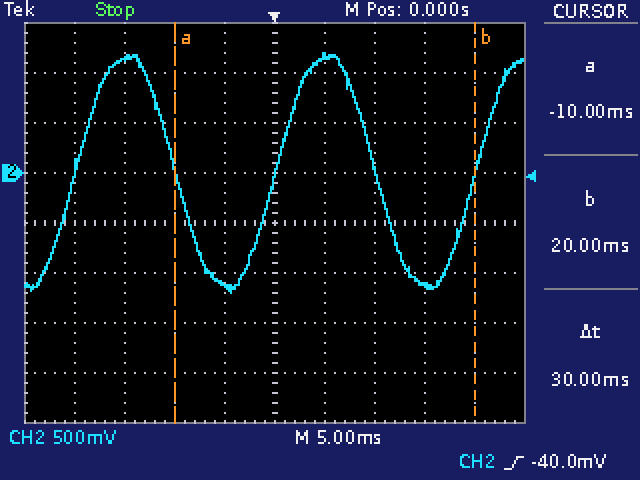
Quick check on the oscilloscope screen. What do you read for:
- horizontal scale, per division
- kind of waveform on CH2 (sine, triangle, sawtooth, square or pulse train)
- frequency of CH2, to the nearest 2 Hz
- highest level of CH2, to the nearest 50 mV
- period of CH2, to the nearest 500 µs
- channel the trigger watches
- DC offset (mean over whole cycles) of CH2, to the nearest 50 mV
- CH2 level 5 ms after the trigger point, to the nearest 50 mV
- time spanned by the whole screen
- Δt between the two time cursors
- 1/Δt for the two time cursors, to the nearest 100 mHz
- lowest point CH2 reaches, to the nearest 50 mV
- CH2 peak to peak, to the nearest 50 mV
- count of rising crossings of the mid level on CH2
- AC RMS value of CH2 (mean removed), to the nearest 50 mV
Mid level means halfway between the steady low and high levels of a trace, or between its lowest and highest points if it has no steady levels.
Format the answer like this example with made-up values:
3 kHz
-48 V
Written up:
5 ms
sine
50 Hz
1.20 V
20.0 ms
CH2
0 mV
1.15 V
50 ms
30 ms
33.3 Hz
-1.20 V
2.40 V
3
850 mV
